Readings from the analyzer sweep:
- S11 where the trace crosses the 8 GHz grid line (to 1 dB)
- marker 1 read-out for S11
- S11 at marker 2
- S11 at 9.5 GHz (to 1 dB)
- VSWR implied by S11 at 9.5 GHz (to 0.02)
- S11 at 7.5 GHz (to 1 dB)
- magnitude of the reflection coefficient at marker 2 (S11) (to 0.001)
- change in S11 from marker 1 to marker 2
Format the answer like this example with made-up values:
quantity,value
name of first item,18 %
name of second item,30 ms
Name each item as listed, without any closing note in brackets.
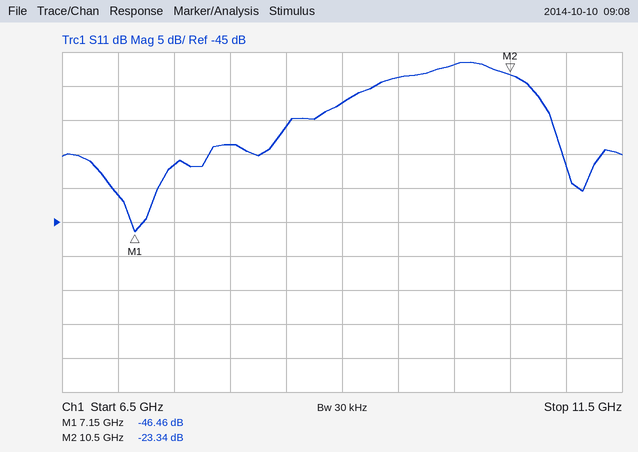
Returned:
quantity,value
S11 where the trace crosses the 8 GHz grid line,-34 dB
marker 1 read-out for S11,-46.46 dB
S11 at marker 2,-23.34 dB
S11 at 9.5 GHz,-24 dB
VSWR implied by S11 at 9.5 GHz,1.14
S11 at 7.5 GHz,-37 dB
magnitude of the reflection coefficient at marker 2 (S11),0.068
change in S11 from marker 1 to marker 2,23.12 dB
